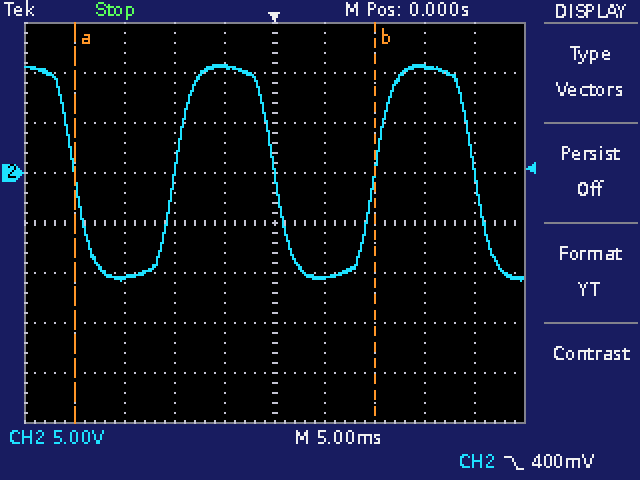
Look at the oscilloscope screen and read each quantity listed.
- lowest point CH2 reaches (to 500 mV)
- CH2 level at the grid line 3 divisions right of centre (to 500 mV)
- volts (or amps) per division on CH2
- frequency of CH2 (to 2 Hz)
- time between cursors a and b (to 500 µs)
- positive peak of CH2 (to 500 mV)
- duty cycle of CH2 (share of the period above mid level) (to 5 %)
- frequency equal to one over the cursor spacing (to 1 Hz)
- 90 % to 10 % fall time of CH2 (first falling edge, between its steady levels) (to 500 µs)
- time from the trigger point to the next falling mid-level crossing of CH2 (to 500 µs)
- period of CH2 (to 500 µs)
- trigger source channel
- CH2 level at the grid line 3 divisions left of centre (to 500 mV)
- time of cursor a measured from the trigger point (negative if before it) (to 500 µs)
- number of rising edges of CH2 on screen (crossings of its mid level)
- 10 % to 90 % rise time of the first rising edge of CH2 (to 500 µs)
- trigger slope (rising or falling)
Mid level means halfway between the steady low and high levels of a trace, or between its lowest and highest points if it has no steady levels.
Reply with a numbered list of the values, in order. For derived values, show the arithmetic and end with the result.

1. -11.0 V
2. 10.5 V
3. 5 V
4. 1 / 20.0 ms ≈ 50 Hz
5. 30.0 ms
6. 11.0 V
7. 50 %
8. 1 / 30.0 ms ≈ 33 Hz
9. 3.5 ms
10. 20.0 ms
11. 20.0 ms
12. CH2
13. -10.5 V
14. -20.0 ms
15. 2
16. 3.5 ms
17. falling
